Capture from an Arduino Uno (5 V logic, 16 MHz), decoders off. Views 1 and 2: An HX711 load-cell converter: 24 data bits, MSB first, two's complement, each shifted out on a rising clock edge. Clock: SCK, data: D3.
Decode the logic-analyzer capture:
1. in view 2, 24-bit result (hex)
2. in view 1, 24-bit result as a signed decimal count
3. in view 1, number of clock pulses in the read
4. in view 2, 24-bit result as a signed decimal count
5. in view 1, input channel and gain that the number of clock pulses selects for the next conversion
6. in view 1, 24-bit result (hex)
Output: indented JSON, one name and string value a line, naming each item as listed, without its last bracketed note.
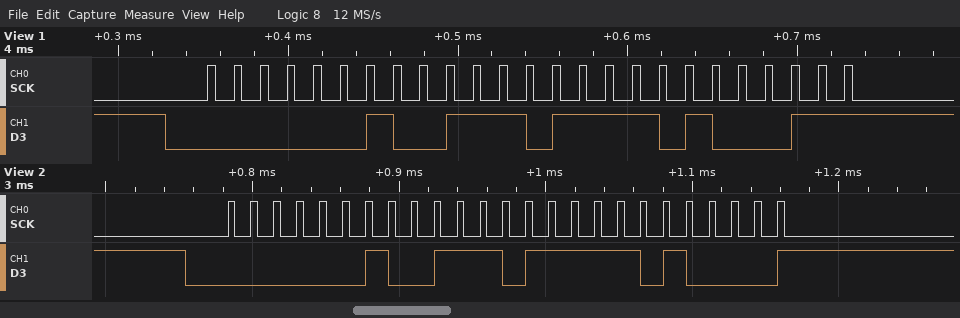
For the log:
{
  "in view 2, 24-bit result": "0x0277D0",
  "in view 1, 24-bit result as a signed decimal count": "161699",
  "in view 1, number of clock pulses in the read": "25",
  "in view 2, 24-bit result as a signed decimal count": "161744",
  "in view 1, input channel and gain that the number of clock pulses selects for the next conversion": "channel A, gain 128",
  "in view 1, 24-bit result": "0x0277A3"
}
